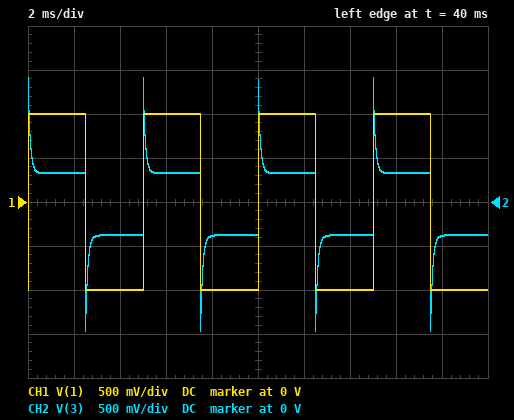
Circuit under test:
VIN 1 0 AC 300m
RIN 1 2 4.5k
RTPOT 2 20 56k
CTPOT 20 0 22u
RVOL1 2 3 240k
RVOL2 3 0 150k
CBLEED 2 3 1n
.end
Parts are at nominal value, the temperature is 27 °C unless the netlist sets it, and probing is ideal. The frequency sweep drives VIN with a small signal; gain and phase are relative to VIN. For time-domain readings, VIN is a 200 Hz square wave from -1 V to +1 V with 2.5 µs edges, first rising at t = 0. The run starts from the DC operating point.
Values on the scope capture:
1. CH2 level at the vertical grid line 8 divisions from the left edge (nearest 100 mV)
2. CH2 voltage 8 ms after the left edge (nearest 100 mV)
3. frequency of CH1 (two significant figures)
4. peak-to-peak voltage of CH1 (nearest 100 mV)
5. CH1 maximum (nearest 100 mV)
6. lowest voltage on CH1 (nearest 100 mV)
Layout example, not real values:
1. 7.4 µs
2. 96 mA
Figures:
1. 300 mV
2. -400 mV
3. 200 Hz
4. 2.0 V
5. 1.0 V
6. -1.0 V
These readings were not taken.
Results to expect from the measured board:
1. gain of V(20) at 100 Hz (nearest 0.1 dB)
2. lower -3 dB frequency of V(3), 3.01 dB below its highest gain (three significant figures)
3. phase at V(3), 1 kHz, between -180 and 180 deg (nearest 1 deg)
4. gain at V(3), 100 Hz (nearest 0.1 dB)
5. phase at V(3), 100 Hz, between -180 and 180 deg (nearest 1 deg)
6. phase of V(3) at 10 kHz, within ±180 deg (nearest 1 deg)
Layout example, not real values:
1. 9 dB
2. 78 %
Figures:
1. -58.5 dB
2. 1.41 kHz
3. 26 deg
4. -9.0 dB
5. 5 deg
6. 6 deg
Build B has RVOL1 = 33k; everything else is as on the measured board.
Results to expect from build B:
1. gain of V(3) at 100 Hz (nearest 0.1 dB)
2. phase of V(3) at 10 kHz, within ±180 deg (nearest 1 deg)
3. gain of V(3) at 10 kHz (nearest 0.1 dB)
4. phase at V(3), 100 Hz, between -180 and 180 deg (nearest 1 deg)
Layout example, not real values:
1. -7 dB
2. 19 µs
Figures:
1. -2.6 dB
2. 5 deg
3. -1.3 dB
4. 0 deg
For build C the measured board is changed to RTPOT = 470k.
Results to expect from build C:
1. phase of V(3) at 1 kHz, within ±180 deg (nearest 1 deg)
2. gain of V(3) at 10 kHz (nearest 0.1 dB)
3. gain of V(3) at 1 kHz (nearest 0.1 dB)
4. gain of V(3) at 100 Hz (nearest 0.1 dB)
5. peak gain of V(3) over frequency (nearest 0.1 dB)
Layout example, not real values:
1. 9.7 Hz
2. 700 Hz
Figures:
1. 26 deg
2. -0.4 dB
3. -4.6 dB
4. -8.4 dB
5. -0.3 dB
